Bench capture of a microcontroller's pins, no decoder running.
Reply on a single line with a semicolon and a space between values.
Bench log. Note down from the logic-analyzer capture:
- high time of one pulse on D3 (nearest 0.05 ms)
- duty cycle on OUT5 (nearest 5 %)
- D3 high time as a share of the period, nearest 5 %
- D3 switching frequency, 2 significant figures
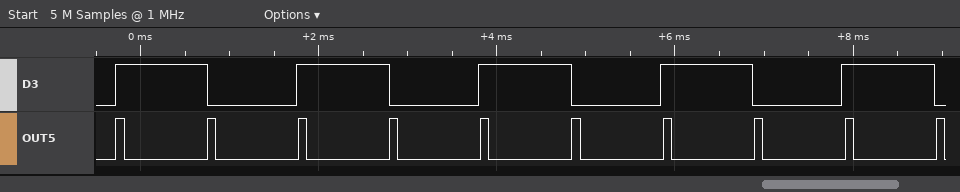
1.05 ms; 10 %; 50 %; 490 Hz
